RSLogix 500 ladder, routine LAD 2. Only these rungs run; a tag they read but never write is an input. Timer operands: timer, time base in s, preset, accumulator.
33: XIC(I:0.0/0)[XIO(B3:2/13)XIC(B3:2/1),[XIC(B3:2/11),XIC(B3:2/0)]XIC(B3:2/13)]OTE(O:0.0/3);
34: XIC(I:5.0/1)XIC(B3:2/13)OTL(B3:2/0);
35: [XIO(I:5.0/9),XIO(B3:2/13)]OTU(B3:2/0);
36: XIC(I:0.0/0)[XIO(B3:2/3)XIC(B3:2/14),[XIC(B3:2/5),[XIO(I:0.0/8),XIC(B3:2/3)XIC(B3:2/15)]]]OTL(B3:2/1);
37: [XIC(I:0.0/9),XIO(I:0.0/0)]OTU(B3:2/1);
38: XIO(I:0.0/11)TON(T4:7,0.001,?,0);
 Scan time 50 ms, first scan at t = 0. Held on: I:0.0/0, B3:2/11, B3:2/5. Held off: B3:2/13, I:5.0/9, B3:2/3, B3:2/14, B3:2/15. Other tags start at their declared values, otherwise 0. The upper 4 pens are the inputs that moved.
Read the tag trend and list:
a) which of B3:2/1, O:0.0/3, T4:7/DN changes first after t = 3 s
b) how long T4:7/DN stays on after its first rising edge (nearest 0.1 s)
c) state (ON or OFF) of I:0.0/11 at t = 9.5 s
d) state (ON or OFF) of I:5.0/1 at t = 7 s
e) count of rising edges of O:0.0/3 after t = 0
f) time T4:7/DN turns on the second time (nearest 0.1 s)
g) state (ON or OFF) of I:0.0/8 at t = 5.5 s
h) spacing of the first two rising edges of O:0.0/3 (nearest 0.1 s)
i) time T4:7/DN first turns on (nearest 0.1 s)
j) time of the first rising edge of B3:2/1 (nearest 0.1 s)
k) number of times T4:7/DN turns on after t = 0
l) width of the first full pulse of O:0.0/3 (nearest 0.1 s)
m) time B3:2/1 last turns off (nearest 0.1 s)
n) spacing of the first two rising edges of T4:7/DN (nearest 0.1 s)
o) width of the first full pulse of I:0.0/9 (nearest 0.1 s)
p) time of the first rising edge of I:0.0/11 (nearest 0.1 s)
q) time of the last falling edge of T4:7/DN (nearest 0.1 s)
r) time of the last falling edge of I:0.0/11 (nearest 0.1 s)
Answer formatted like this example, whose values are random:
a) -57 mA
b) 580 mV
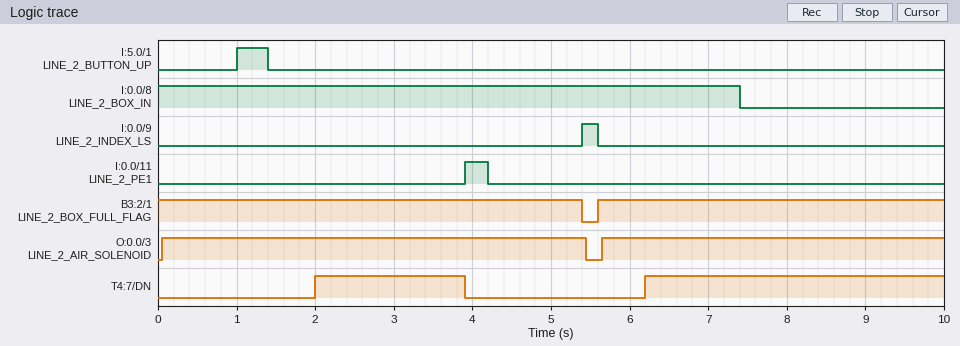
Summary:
a) T4:7/DN
b) 1.9 s
c) OFF
d) OFF
e) 2
f) 6.2 s
g) ON
h) 5.6 s
i) 2.0 s
j) 5.6 s
k) 2
l) 5.4 s
m) 5.4 s
n) 4.2 s
o) 0.2 s
p) 3.9 s
q) 3.9 s
r) 4.2 s
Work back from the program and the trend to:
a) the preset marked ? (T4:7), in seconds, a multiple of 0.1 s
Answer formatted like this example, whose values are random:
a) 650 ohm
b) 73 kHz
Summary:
a) 2.0 s
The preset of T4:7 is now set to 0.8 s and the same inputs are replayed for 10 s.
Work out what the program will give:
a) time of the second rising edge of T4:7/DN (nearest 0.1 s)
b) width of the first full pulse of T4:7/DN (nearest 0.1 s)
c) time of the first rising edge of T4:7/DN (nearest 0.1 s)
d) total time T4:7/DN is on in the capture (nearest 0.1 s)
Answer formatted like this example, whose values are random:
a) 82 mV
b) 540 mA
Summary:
a) 5.0 s
b) 3.1 s
c) 0.8 s
d) 8.1 s
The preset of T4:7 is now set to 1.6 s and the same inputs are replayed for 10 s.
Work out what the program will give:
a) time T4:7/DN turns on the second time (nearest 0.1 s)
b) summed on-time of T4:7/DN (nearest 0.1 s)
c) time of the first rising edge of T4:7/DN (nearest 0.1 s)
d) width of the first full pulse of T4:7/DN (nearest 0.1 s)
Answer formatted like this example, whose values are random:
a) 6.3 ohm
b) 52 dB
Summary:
a) 5.8 s
b) 6.5 s
c) 1.6 s
d) 2.3 s
